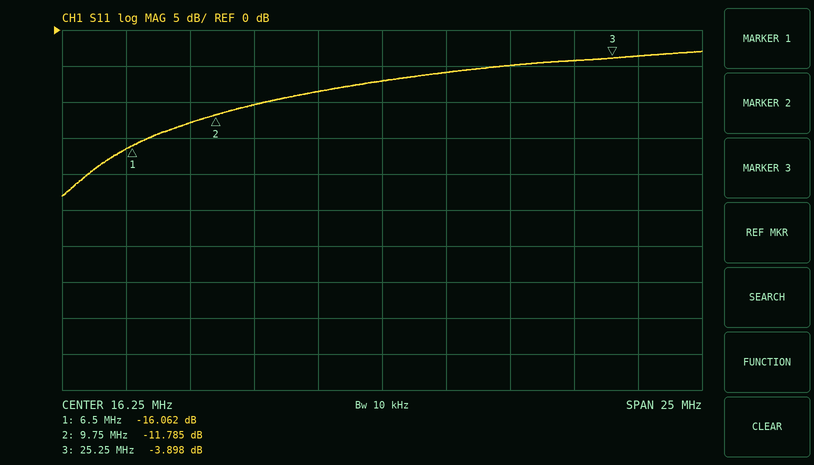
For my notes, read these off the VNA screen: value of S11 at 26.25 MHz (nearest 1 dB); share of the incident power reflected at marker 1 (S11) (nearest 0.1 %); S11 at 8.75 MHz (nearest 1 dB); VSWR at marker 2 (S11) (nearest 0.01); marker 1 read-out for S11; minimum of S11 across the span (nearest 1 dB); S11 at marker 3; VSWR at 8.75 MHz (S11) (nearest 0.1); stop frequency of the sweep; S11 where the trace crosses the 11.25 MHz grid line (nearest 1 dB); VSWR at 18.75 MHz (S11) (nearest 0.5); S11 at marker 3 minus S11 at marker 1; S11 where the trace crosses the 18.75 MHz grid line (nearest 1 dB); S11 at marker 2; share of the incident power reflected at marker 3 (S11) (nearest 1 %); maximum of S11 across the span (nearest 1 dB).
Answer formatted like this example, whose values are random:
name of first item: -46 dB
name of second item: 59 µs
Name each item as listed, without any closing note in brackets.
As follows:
value of S11 at 26.25 MHz: -4 dB
share of the incident power reflected at marker 1 (S11): 2.5 %
S11 at 8.75 MHz: -13 dB
VSWR at marker 2 (S11): 1.69
marker 1 read-out for S11: -16.062 dB
minimum of S11 across the span: -23 dB
S11 at marker 3: -3.898 dB
VSWR at 8.75 MHz (S11): 1.6
stop frequency of the sweep: 28.75 MHz
S11 where the trace crosses the 11.25 MHz grid line: -10 dB
VSWR at 18.75 MHz (S11): 3.0
S11 at marker 3 minus S11 at marker 1: 12.164 dB
S11 where the trace crosses the 18.75 MHz grid line: -6 dB
S11 at marker 2: -11.785 dB
share of the incident power reflected at marker 3 (S11): 41 %
maximum of S11 across the span: -3 dB
